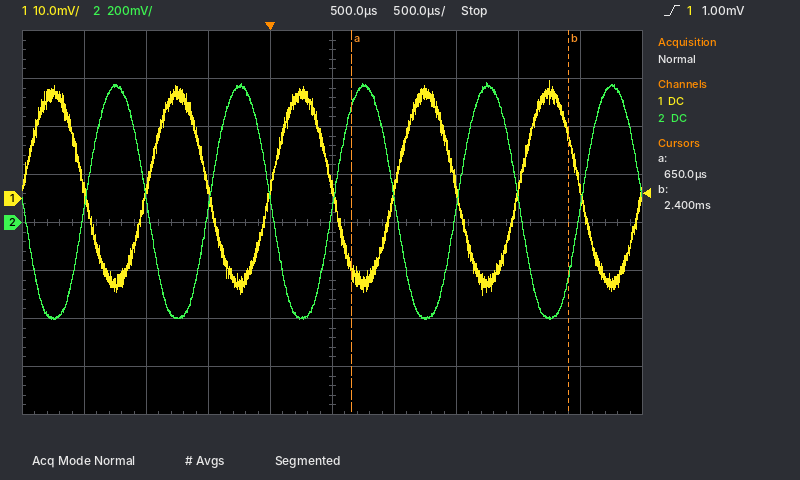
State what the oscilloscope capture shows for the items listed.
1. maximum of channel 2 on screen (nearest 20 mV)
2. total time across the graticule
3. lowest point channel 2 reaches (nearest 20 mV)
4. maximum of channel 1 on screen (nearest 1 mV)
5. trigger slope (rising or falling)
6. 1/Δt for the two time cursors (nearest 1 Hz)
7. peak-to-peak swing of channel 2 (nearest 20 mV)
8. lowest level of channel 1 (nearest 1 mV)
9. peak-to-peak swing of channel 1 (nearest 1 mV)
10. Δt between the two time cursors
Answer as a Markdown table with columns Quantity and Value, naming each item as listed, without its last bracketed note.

| Quantity | Value |
|---|---|
| maximum of channel 2 on screen | 580 mV |
| total time across the graticule | 5 ms |
| lowest point channel 2 reaches | -400 mV |
| maximum of channel 1 on screen | 25 mV |
| trigger slope | rising |
| 1/Δt for the two time cursors | 571 Hz |
| peak-to-peak swing of channel 2 | 980 mV |
| lowest level of channel 1 | -20 mV |
| peak-to-peak swing of channel 1 | 45 mV |
| Δt between the two time cursors | 1.75 ms |
